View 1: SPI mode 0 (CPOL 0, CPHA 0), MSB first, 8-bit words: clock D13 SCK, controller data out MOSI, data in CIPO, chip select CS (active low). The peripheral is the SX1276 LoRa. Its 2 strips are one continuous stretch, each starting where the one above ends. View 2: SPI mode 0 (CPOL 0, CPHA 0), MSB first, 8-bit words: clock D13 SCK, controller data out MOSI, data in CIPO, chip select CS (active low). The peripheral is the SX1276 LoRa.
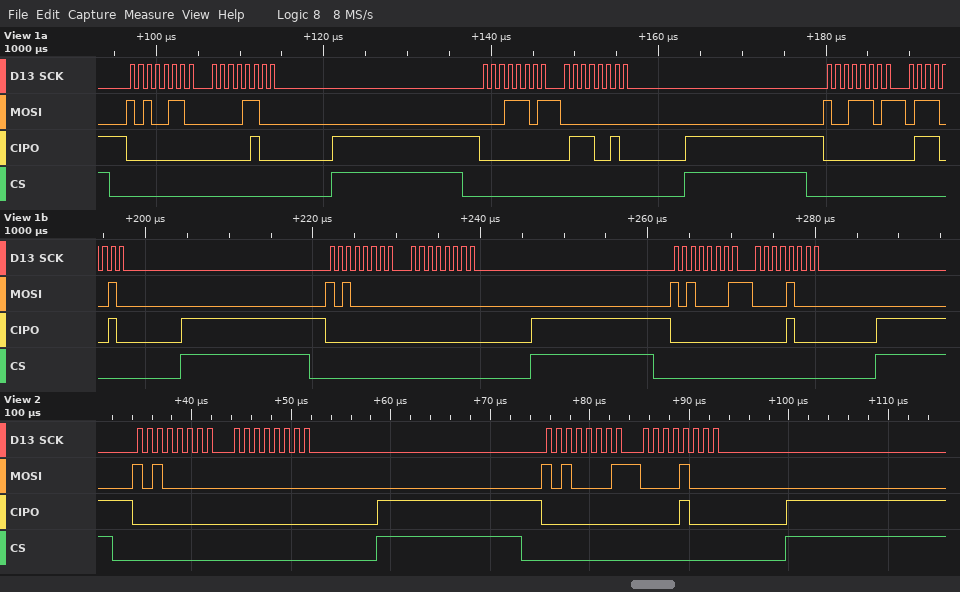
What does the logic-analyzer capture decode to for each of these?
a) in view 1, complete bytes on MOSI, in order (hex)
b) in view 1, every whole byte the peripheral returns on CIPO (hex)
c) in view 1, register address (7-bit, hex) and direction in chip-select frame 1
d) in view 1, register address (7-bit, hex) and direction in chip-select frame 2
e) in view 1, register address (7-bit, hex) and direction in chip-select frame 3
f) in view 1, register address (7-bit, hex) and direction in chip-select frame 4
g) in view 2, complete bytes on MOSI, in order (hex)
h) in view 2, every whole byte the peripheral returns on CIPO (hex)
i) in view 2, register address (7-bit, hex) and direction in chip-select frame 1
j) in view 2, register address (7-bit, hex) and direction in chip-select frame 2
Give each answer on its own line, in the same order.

A6 0C 1D 00 9D 72 A0 00 A1 08
00 04 00 72 00 72 00 00 00 08
0x26 write
0x1D read
0x1D write
0x20 write
A0 00 A1 08
00 00 00 08
0x20 write
0x21 write
